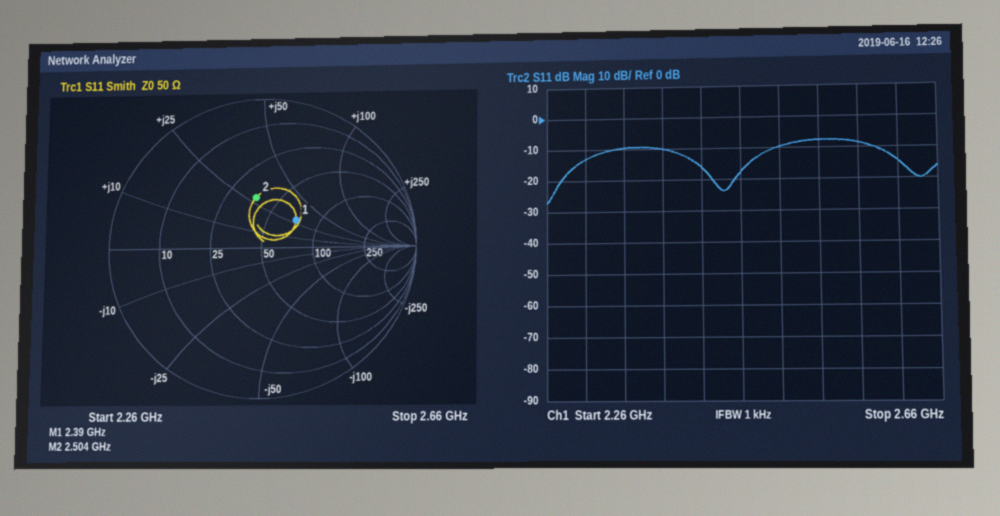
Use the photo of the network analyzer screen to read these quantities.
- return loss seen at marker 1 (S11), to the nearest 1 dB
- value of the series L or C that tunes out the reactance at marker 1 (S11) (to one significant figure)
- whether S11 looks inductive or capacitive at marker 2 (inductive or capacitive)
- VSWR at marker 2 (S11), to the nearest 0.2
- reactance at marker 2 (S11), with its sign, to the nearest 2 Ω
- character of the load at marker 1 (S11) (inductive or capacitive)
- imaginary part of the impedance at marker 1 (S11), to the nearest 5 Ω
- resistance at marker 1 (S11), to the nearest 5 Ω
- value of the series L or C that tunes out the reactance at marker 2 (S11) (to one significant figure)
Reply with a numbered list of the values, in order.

1. 11 dB
2. 2 pF
3. inductive
4. 2.0
5. +28 Ω
6. inductive
7. +30 Ω
8. 70 Ω
9. 2 pF
